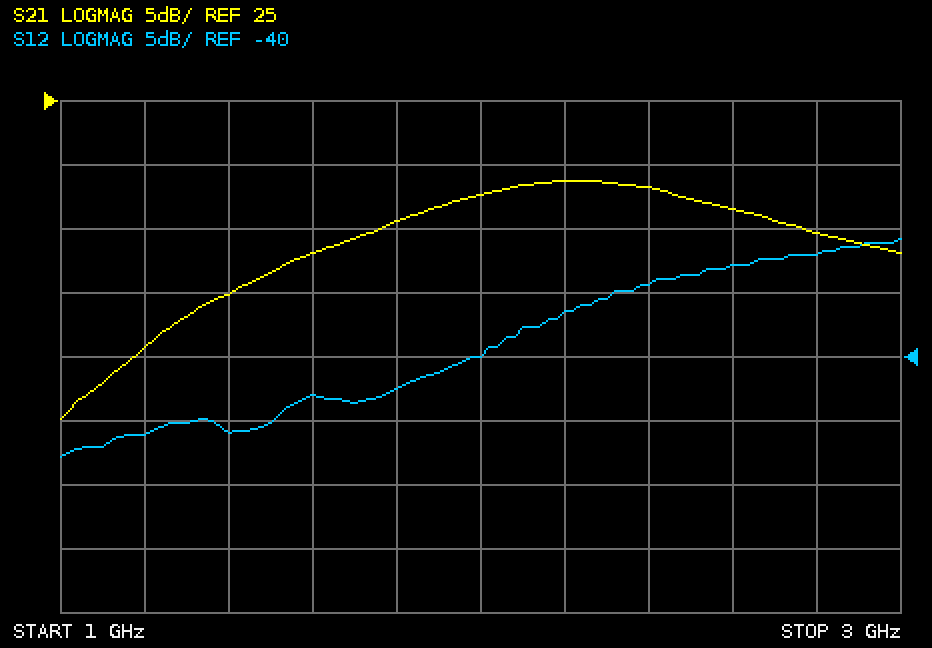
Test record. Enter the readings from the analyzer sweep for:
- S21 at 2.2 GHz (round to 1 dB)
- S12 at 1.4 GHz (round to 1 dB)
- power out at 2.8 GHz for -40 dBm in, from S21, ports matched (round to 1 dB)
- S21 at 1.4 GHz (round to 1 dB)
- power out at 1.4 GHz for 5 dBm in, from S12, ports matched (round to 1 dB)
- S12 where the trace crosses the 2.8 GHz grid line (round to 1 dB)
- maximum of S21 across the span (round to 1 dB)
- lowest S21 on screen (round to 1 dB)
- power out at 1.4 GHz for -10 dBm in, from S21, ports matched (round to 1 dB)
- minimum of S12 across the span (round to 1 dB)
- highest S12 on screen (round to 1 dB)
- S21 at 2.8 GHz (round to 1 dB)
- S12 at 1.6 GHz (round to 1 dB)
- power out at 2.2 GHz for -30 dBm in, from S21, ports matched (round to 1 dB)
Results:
19 dB
-46 dB
-25 dBm
10 dB
-41 dBm
-32 dB
19 dB
0 dB
0 dBm
-48 dB
-31 dB
15 dB
-43 dB
-11 dBm
